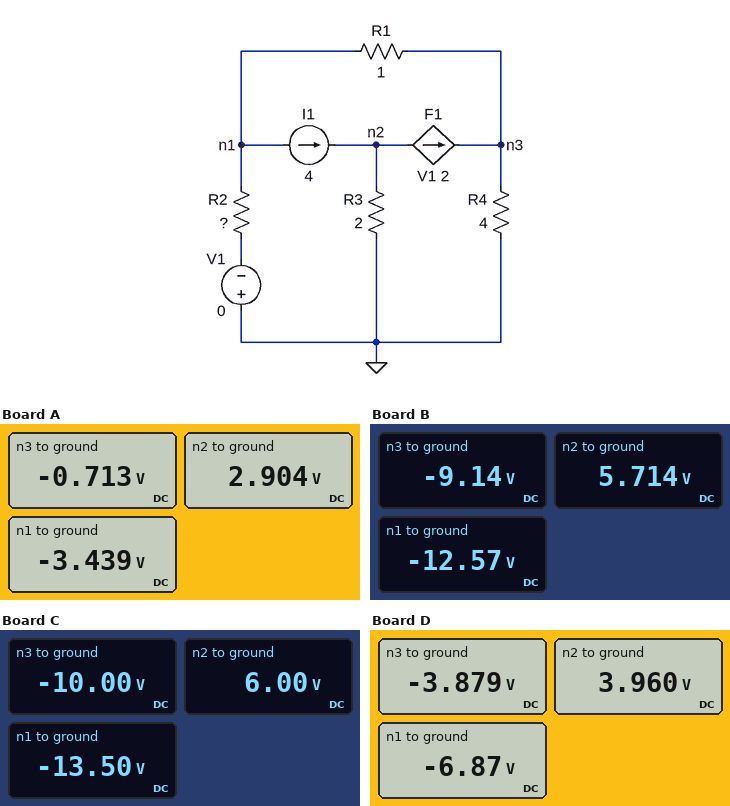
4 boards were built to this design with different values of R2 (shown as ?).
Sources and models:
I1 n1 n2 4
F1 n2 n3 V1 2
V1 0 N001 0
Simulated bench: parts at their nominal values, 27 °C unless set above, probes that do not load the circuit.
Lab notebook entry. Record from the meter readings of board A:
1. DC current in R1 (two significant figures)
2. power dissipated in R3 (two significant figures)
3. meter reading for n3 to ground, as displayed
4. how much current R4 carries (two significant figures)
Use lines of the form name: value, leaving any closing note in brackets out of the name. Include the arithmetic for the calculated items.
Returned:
DC current in R1: (-713 mV - (-3.439 V)) / 1 Ω = 2.7 A
power dissipated in R3: (2.904 V)^2 / 2 Ω = 4.2 W
meter reading for n3 to ground, as displayed: -0.713 V
how much current R4 carries: (0 V - (-713 mV)) / 4 Ω = 180 mA
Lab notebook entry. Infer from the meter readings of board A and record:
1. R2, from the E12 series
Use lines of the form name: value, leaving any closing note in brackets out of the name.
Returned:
R2, from the E12 series: 2.7 Ω
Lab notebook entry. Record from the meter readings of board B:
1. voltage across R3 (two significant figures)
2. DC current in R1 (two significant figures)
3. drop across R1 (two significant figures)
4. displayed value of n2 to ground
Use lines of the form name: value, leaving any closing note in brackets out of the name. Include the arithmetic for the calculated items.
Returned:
voltage across R3: 5.714 V = 5.7 V
DC current in R1: (-9.14 V - (-12.57 V)) / 1 Ω = 3.4 A
drop across R1: -9.14 V - (-12.57 V) = 3.4 V
displayed value of n2 to ground: 5.714 V
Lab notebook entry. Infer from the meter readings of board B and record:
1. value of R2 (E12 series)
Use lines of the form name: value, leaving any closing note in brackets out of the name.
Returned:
value of R2: 22 Ω
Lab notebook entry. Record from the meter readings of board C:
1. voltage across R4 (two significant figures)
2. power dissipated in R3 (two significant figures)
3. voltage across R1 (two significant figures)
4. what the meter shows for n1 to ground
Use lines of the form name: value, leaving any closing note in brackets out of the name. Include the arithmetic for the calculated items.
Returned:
voltage across R4: 0 V - (-10 V) = 10 V
power dissipated in R3: (6 V)^2 / 2 Ω = 18 W
voltage across R1: -10 V - (-13.5 V) = 3.5 V
what the meter shows for n1 to ground: -13.50 V
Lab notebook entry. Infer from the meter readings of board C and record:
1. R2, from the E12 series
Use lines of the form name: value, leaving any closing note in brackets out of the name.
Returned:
R2, from the E12 series: 27 Ω
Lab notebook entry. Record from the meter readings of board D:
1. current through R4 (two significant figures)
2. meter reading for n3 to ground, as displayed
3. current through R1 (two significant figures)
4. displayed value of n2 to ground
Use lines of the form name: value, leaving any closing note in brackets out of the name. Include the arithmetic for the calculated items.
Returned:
current through R4: (0 V - (-3.879 V)) / 4 Ω = 970 mA
meter reading for n3 to ground, as displayed: -3.879 V
current through R1: (-3.879 V - (-6.87 V)) / 1 Ω = 3.0 A
displayed value of n2 to ground: 3.960 V
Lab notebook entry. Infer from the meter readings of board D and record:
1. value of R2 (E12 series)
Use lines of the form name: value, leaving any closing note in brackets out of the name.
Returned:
value of R2: 6.8 Ω
